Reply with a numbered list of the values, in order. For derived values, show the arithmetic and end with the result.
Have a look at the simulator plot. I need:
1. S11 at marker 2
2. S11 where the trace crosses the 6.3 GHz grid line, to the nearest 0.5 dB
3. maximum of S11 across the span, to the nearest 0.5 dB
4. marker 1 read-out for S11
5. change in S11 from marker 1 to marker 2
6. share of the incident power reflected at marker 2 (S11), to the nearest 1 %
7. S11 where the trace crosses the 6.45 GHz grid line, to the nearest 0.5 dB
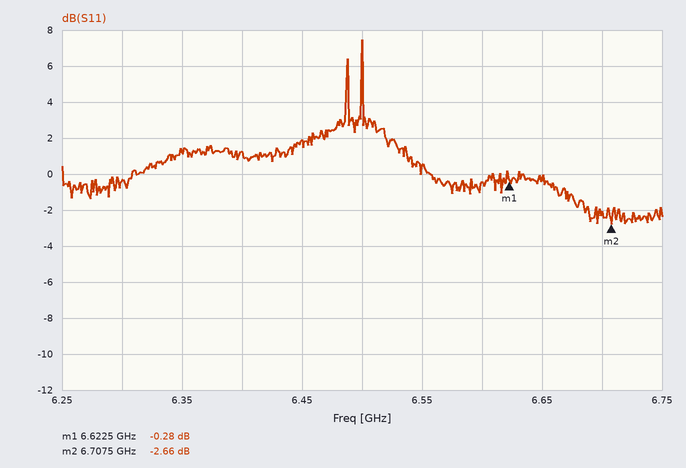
1. -2.66 dB
2. -0.5 dB
3. 7.5 dB
4. -0.28 dB
5. -2.66 − (-0.28) = -2.38 dB
6. 10^(-2.66/10) ≈ 54 %
7. 2.0 dB
